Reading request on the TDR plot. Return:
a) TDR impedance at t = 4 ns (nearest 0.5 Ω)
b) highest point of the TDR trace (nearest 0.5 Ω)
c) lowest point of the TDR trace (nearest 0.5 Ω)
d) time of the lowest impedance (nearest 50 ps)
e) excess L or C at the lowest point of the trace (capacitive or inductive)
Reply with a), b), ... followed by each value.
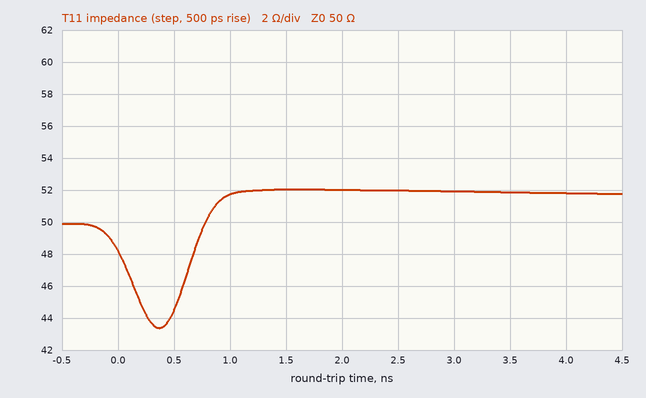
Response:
a) 52.0 Ω
b) 52.0 Ω
c) 43.5 Ω
d) 350 ps
e) capacitive
